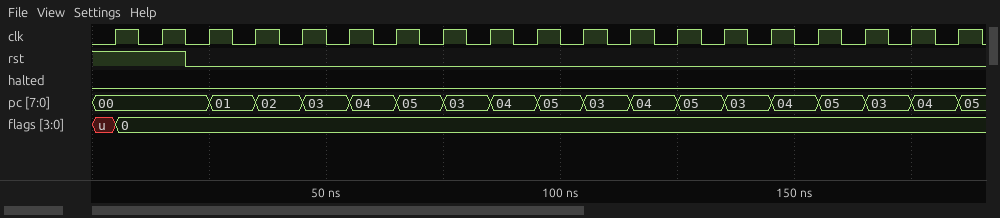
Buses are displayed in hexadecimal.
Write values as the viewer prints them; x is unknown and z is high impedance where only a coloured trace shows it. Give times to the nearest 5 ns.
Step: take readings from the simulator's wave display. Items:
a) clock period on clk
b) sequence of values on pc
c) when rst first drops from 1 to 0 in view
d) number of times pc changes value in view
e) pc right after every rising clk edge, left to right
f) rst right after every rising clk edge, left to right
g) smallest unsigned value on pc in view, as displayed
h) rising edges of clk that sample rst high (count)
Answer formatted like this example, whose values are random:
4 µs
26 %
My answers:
10 ns
00, 01, 02, 03, 04, 05, 03, 04, 05, 03, 04, 05, 03, 04, 05, 03, 04, 05
20 ns
17
00, 00, 01, 02, 03, 04, 05, 03, 04, 05, 03, 04, 05, 03, 04, 05, 03, 04, 05
1 1 0 0 0 0 0 0 0 0 0 0 0 0 0 0 0 0 0
00
2
